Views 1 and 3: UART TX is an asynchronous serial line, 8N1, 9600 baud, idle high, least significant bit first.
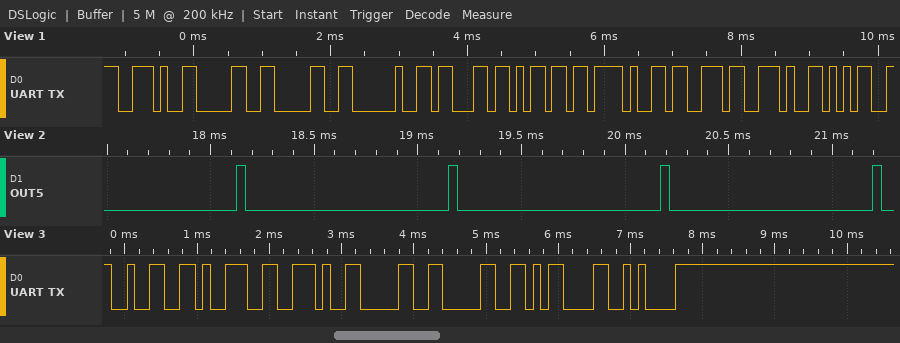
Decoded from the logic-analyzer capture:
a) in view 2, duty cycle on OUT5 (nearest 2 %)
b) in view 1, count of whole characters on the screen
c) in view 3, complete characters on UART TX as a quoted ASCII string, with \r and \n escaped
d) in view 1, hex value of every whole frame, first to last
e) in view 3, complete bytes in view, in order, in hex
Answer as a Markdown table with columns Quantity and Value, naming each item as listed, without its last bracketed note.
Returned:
| Quantity | Value |
|---|---|
| in view 2, duty cycle on OUT5 | 4 % |
| in view 1, count of whole characters on the screen | 10 |
| in view 3, complete characters on UART TX as a quoted ASCII string, with \r and \n escaped | "29.00\r\n" |
| in view 1, hex value of every whole frame, first to last | 2E 30 30 20 63 6D 2F 73 2E 35 |
| in view 3, complete bytes in view, in order, in hex | 32 39 2E 30 30 0D 0A |
